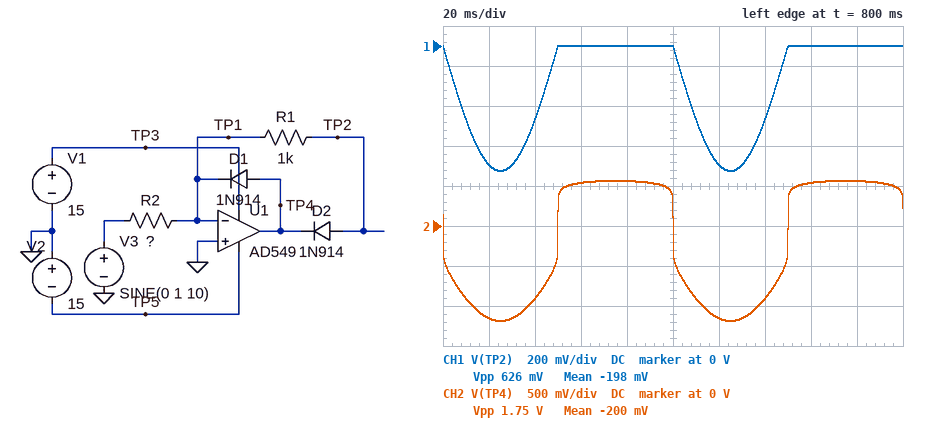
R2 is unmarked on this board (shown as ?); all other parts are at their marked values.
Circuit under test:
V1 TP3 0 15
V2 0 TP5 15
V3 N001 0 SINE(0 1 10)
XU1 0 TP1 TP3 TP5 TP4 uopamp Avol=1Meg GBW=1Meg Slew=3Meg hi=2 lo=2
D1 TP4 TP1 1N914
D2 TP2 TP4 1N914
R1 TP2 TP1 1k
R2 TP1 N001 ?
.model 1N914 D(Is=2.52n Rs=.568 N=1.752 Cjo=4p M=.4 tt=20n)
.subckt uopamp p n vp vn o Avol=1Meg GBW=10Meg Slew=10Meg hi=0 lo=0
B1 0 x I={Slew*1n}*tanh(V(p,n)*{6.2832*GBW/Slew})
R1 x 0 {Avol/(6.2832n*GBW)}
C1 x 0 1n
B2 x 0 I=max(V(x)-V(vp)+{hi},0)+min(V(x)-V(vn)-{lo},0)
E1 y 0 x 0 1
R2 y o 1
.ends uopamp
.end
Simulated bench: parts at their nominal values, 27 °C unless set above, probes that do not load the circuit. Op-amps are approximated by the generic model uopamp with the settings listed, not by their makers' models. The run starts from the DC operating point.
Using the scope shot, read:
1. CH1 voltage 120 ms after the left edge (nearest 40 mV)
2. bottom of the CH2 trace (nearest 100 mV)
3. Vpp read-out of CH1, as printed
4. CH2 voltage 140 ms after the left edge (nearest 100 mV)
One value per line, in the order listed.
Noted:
-600 mV
-1.2 V
626 mV
-900 mV
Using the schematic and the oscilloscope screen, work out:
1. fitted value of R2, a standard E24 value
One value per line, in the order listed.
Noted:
1.6 kΩ
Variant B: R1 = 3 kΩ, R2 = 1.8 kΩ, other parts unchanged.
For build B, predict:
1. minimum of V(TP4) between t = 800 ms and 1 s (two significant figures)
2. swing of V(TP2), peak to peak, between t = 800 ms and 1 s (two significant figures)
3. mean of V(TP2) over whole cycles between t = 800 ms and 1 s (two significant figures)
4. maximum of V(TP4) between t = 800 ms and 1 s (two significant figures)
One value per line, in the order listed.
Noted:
-2.2 V
1.7 V
-530 mV
560 mV
